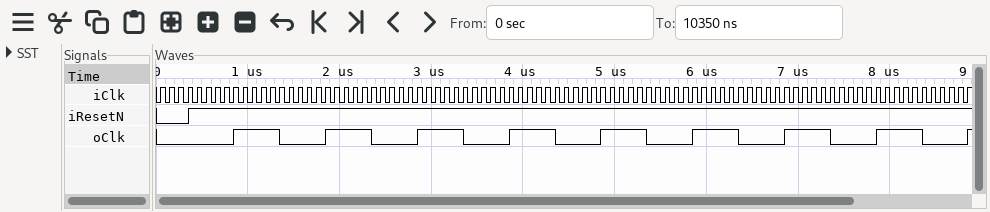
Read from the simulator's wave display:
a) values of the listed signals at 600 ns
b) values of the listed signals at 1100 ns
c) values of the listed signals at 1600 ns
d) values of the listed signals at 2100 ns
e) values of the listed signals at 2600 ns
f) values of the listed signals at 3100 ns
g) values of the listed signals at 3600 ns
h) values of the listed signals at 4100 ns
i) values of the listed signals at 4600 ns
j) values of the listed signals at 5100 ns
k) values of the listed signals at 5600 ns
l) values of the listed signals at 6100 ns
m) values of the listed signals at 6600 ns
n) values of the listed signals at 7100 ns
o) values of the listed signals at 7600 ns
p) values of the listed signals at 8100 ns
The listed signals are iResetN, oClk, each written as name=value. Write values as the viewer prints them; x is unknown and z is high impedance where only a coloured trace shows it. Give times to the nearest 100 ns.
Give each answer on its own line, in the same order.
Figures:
iResetN=1, oClk=0
iResetN=1, oClk=1
iResetN=1, oClk=0
iResetN=1, oClk=1
iResetN=1, oClk=0
iResetN=1, oClk=1
iResetN=1, oClk=0
iResetN=1, oClk=1
iResetN=1, oClk=0
iResetN=1, oClk=1
iResetN=1, oClk=0
iResetN=1, oClk=1
iResetN=1, oClk=0
iResetN=1, oClk=1
iResetN=1, oClk=0
iResetN=1, oClk=1
